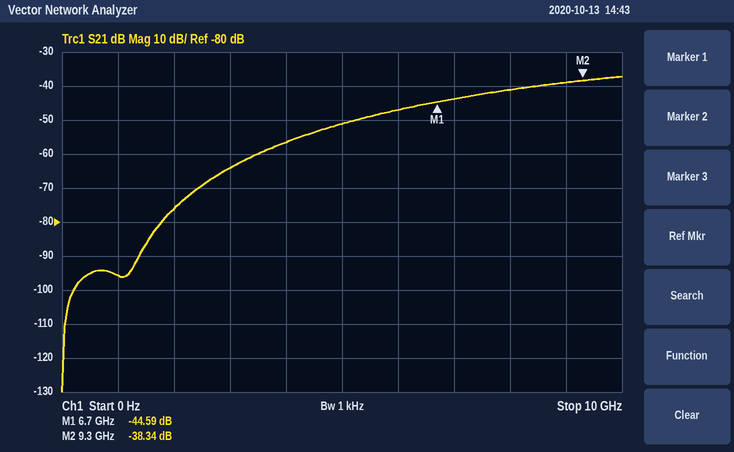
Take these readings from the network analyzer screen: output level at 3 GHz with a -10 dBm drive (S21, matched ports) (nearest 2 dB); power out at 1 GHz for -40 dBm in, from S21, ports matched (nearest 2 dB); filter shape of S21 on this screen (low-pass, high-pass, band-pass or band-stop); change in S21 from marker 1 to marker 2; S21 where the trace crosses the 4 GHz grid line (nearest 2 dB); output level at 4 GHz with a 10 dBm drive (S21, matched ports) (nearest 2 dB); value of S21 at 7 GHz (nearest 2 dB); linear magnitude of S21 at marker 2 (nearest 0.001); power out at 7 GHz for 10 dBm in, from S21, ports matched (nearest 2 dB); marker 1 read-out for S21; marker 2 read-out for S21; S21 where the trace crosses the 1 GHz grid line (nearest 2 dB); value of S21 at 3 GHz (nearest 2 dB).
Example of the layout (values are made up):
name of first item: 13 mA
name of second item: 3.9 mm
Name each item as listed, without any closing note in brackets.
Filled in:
output level at 3 GHz with a -10 dBm drive (S21, matched ports): -74 dBm
power out at 1 GHz for -40 dBm in, from S21, ports matched: -136 dBm
filter shape of S21 on this screen: high-pass
change in S21 from marker 1 to marker 2: 6.25 dB
S21 where the trace crosses the 4 GHz grid line: -56 dB
output level at 4 GHz with a 10 dBm drive (S21, matched ports): -46 dBm
value of S21 at 7 GHz: -44 dB
linear magnitude of S21 at marker 2: 0.012
power out at 7 GHz for 10 dBm in, from S21, ports matched: -34 dBm
marker 1 read-out for S21: -44.59 dB
marker 2 read-out for S21: -38.34 dB
S21 where the trace crosses the 1 GHz grid line: -96 dB
value of S21 at 3 GHz: -64 dB
